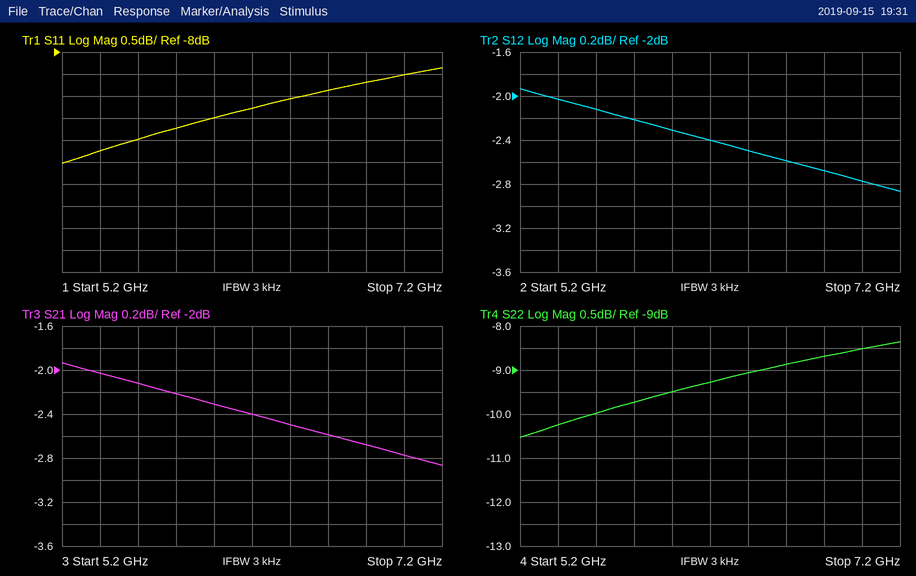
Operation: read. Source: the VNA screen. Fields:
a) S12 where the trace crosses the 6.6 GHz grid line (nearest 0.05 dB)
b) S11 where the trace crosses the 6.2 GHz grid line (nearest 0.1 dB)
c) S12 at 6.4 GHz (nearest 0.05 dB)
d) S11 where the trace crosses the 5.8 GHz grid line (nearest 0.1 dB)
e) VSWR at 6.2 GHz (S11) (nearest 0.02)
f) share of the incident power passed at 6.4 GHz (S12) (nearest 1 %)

-2.60 dB
-9.3 dB
-2.50 dB
-9.7 dB
2.04
56 %
